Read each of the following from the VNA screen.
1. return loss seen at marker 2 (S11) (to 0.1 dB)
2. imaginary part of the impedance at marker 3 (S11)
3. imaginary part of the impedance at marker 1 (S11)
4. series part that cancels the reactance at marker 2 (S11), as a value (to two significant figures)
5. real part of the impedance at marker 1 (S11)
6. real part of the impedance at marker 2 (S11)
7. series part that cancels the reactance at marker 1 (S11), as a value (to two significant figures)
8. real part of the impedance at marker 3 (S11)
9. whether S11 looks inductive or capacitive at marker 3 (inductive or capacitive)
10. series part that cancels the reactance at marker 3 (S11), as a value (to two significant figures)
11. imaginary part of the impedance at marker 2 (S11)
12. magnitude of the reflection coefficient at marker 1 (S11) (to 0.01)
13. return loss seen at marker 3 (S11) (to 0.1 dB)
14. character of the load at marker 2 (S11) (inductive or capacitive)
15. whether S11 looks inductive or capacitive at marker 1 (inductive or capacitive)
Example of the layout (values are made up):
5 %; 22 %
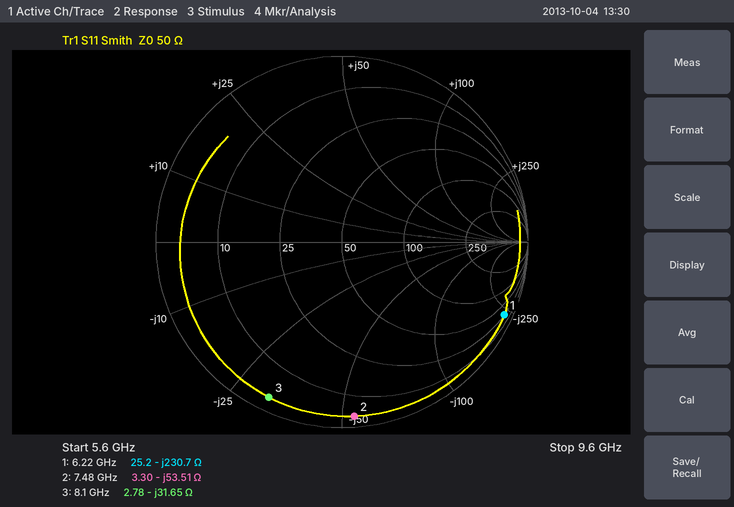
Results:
0.5 dB; -31.65 Ω; -230.7 Ω; 1.1 nH; 25.2 Ω; 3.30 Ω; 5.9 nH; 2.78 Ω; capacitive; 620 pH; -53.51 Ω; 0.96; 0.7 dB; capacitive; capacitive
